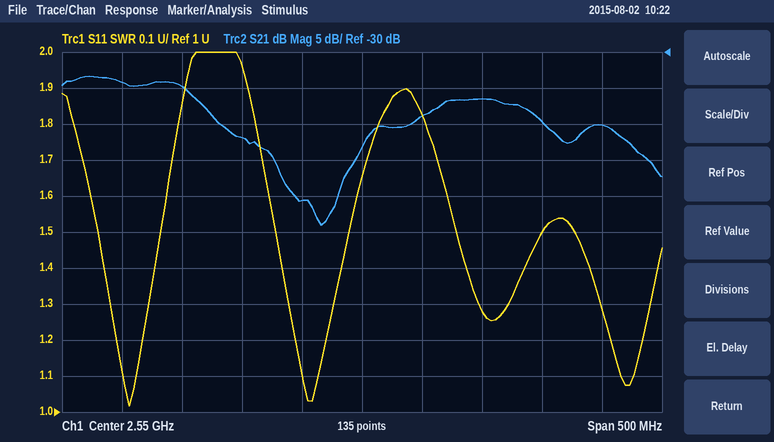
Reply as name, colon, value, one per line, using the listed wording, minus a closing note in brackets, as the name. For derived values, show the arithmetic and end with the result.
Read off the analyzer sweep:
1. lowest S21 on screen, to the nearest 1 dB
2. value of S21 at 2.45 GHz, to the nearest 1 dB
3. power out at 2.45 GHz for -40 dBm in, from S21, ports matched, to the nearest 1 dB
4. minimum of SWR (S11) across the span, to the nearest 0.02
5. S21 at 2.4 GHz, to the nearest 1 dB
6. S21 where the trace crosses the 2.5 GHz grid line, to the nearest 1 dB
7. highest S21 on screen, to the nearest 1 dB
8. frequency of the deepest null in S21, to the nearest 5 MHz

lowest S21 on screen, to the nearest 1 dB: -54 dB
value of S21 at 2.45 GHz, to the nearest 1 dB: -42 dB
power out at 2.45 GHz for -40 dBm in, from S21, ports matched, to the nearest 1 dB: -40 dBm + (-42 dB) = -82 dBm
minimum of SWR (S11) across the span, to the nearest 0.02: 1.02
S21 at 2.4 GHz, to the nearest 1 dB: -35 dB
S21 where the trace crosses the 2.5 GHz grid line, to the nearest 1 dB: -51 dB
highest S21 on screen, to the nearest 1 dB: -33 dB
frequency of the deepest null in S21, to the nearest 5 MHz: 2.515 GHz
